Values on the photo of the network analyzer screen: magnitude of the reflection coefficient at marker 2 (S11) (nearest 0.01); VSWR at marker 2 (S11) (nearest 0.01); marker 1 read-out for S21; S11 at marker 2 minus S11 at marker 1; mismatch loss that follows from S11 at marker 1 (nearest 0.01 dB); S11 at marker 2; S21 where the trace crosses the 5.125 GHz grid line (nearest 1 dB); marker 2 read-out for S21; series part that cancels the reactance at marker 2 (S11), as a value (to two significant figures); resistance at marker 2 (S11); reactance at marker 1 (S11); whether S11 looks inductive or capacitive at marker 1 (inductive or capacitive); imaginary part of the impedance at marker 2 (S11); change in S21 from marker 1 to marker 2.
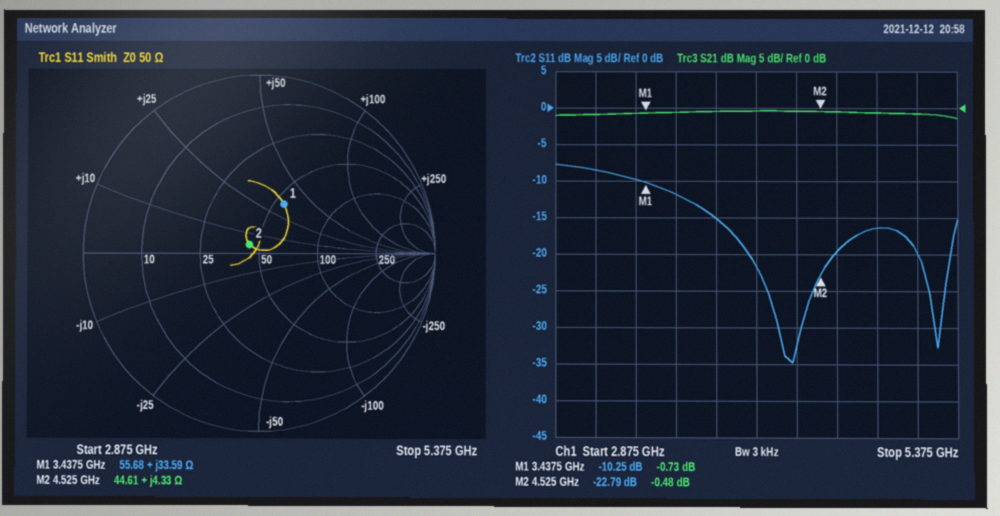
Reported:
0.07
1.16
-0.73 dB
-12.54 dB
0.43 dB
-22.79 dB
-1 dB
-0.48 dB
8.1 pF
44.61 Ω
+33.59 Ω
inductive
+4.33 Ω
0.25 dB
